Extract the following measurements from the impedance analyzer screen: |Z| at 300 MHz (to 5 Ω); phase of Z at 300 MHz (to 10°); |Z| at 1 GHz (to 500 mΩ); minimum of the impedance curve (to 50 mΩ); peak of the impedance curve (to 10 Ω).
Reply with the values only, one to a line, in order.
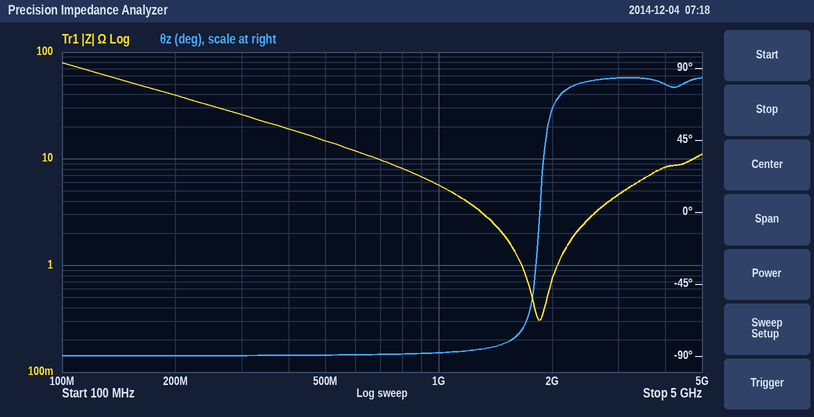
25 Ω
-90°
5.5 Ω
300 mΩ
80 Ω
